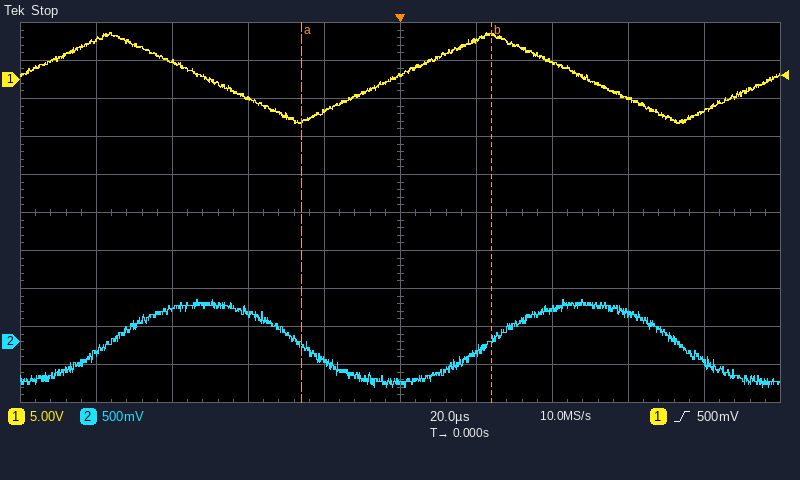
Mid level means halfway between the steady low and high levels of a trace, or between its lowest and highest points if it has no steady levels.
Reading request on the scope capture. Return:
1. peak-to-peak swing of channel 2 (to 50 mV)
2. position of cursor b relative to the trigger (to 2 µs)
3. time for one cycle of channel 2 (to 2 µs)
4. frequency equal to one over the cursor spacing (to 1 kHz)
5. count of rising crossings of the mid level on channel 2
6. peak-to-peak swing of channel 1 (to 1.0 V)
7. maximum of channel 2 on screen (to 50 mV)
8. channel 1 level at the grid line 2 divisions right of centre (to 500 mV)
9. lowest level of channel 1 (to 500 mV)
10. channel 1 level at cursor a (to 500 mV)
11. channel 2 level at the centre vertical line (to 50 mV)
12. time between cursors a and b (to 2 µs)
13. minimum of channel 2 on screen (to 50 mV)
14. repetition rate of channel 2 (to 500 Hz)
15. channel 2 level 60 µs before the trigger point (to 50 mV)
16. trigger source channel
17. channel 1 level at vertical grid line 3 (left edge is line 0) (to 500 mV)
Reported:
1.15 V
+24 µs
100 µs
20 kHz
2
12.0 V
550 mV
2.5 V
-6.0 V
-5.5 V
-500 mV
50 µs
-600 mV
10.0 kHz
450 mV
channel 1
-2.5 V
